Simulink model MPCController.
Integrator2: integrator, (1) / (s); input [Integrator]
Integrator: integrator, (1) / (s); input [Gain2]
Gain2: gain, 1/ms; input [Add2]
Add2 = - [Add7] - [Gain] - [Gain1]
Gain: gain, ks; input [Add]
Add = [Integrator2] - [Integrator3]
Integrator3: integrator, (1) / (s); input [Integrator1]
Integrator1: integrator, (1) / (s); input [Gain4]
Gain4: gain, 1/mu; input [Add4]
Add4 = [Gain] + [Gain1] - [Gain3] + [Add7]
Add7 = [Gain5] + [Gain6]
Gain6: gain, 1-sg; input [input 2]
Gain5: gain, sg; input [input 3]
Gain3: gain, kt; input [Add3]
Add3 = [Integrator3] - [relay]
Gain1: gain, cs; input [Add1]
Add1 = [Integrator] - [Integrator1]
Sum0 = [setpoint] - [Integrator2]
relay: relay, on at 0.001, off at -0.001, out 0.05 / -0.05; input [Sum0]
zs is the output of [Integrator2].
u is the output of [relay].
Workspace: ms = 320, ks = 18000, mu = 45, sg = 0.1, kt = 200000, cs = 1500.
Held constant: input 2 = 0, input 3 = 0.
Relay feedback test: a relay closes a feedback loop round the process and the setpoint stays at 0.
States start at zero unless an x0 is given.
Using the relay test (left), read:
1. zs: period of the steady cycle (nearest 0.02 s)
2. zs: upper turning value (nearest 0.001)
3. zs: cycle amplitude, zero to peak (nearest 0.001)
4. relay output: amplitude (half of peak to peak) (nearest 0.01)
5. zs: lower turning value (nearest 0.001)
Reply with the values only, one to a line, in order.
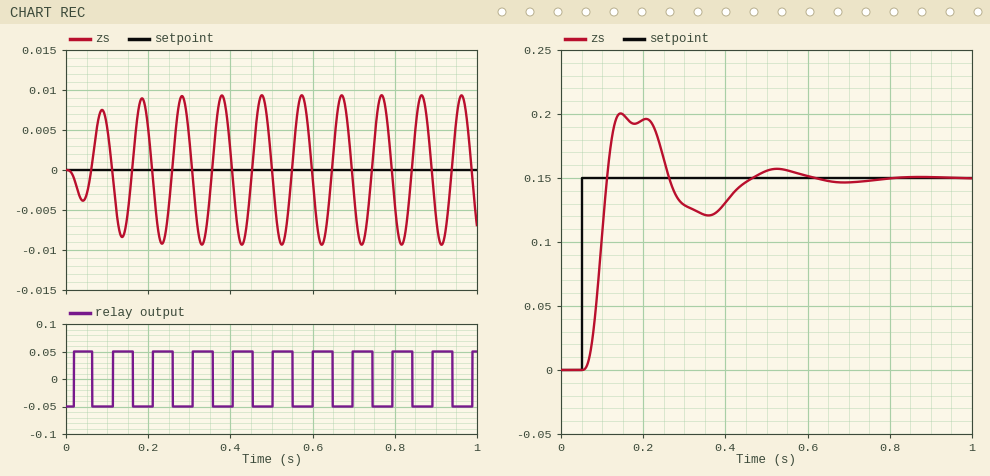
0.10 s
0.009
0.009
0.05
-0.009
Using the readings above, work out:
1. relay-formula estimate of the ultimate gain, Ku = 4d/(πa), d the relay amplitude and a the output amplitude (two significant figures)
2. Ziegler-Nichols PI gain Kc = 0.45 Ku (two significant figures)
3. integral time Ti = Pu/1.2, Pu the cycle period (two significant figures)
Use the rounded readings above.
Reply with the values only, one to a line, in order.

7.1
3.2
0.083 s
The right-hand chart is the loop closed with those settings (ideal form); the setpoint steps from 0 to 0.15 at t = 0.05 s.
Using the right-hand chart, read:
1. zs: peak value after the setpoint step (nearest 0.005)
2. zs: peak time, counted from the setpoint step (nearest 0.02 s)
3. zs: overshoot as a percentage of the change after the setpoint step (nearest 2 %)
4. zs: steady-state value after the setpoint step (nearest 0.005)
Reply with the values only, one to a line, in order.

0.200
0.10 s
34 %
0.150
